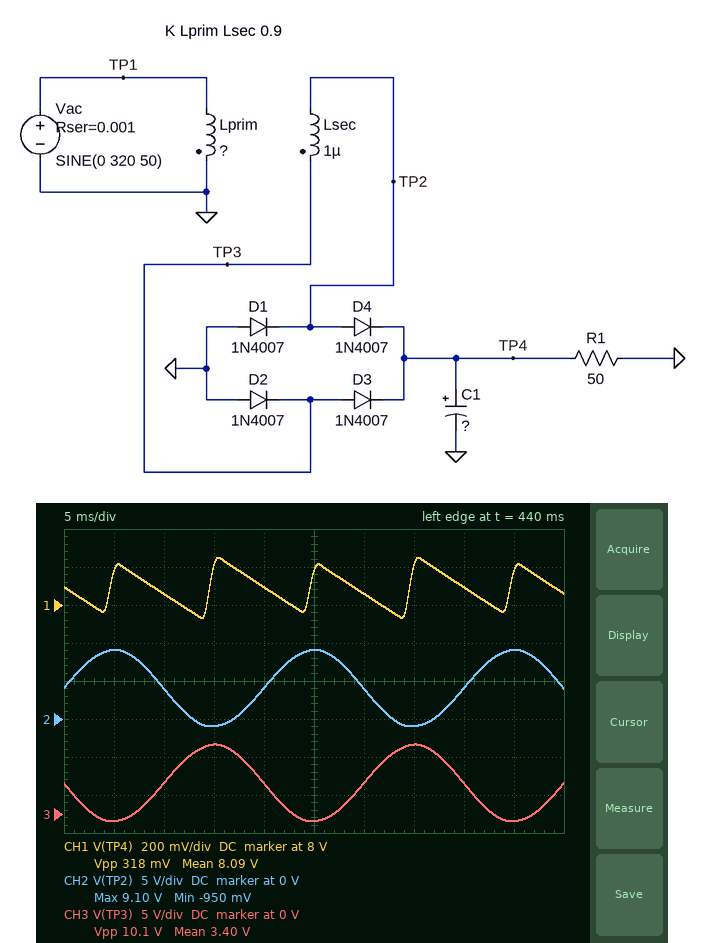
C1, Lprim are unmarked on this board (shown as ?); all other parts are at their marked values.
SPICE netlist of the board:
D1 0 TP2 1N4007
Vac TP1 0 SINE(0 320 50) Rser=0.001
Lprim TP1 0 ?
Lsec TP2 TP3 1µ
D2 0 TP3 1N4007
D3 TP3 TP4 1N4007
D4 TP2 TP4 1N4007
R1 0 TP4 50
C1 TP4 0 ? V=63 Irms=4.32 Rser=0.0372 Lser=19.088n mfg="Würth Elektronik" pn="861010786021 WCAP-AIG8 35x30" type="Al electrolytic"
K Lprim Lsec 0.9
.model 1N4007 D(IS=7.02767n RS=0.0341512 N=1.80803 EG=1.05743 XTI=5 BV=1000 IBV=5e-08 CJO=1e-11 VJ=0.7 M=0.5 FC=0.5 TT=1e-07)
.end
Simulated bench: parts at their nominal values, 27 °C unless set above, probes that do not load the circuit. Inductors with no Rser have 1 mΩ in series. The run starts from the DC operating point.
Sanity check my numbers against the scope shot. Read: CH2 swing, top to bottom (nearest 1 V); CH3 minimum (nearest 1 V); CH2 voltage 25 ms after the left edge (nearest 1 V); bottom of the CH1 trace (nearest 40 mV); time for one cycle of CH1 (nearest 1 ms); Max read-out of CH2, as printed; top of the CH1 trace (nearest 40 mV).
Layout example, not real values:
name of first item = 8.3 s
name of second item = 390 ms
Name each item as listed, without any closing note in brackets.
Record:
CH2 swing, top to bottom = 10 V
CH3 minimum = -1 V
CH2 voltage 25 ms after the left edge = 9 V
bottom of the CH1 trace = 7.92 V
time for one cycle of CH1 = 10 ms
Max read-out of CH2, as printed = 9.10 V
top of the CH1 trace = 8.24 V
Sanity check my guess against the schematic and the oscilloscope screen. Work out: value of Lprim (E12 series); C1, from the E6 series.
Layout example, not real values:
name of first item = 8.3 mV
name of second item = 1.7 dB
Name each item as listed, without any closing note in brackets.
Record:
value of Lprim = 820 µH
C1, from the E6 series = 4.7 mF
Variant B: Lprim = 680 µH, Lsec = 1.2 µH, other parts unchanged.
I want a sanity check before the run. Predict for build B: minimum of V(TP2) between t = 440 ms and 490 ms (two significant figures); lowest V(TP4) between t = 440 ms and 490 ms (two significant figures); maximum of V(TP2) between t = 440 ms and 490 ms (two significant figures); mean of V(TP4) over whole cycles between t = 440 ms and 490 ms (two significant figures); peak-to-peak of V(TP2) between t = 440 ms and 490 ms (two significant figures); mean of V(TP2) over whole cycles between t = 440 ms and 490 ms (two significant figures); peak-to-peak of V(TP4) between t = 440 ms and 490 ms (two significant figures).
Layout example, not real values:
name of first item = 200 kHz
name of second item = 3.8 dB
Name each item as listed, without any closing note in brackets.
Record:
minimum of V(TP2) between t = 440 ms and 490 ms = -980 mV
lowest V(TP4) between t = 440 ms and 490 ms = 9.9 V
maximum of V(TP2) between t = 440 ms and 490 ms = 11 V
mean of V(TP4) over whole cycles between t = 440 ms and 490 ms = 10 V
peak-to-peak of V(TP2) between t = 440 ms and 490 ms = 12 V
mean of V(TP2) over whole cycles between t = 440 ms and 490 ms = 5.0 V
peak-to-peak of V(TP4) between t = 440 ms and 490 ms = 400 mV
